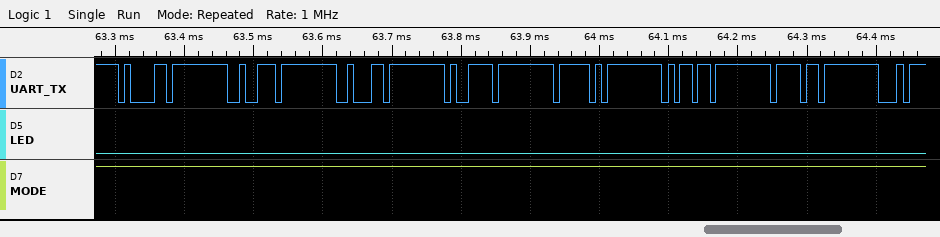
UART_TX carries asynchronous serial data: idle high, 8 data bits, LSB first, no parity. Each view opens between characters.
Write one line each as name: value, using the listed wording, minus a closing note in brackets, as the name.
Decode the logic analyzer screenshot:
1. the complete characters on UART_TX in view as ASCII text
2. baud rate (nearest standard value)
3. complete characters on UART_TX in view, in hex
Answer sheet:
the complete characters on UART_TX in view as ASCII text: "arby_mo"
baud rate: 115200 baud
complete characters on UART_TX in view, in hex: 61, 72, 62, 79, 5F, 6D, 6F
